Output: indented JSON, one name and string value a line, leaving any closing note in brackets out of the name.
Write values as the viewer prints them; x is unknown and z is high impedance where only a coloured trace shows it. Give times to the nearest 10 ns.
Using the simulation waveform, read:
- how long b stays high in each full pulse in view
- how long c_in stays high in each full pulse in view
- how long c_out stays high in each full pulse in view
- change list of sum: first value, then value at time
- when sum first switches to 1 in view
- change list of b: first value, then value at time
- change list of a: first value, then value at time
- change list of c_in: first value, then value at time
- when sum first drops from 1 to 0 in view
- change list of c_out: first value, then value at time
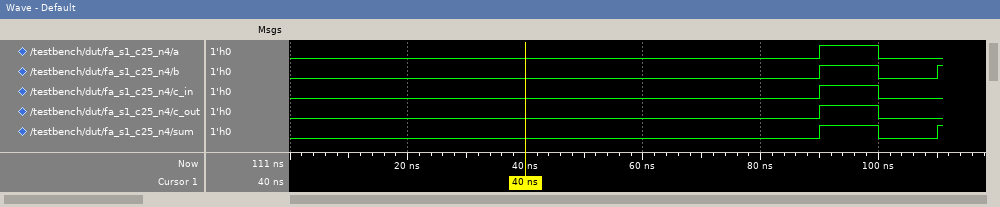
{
  "how long b stays high in each full pulse in view": "10 ns",
  "how long c_in stays high in each full pulse in view": "10 ns",
  "how long c_out stays high in each full pulse in view": "10 ns",
  "change list of sum: first value, then value at time": "0, 1 at 90 ns, 0 at 100 ns, 1 at 110 ns",
  "when sum first switches to 1 in view": "90 ns",
  "change list of b: first value, then value at time": "0, 1 at 90 ns, 0 at 100 ns, 1 at 110 ns",
  "change list of a: first value, then value at time": "0, 1 at 90 ns, 0 at 100 ns",
  "change list of c_in: first value, then value at time": "0, 1 at 90 ns, 0 at 100 ns",
  "when sum first drops from 1 to 0 in view": "100 ns",
  "change list of c_out: first value, then value at time": "0, 1 at 90 ns, 0 at 100 ns"
}
